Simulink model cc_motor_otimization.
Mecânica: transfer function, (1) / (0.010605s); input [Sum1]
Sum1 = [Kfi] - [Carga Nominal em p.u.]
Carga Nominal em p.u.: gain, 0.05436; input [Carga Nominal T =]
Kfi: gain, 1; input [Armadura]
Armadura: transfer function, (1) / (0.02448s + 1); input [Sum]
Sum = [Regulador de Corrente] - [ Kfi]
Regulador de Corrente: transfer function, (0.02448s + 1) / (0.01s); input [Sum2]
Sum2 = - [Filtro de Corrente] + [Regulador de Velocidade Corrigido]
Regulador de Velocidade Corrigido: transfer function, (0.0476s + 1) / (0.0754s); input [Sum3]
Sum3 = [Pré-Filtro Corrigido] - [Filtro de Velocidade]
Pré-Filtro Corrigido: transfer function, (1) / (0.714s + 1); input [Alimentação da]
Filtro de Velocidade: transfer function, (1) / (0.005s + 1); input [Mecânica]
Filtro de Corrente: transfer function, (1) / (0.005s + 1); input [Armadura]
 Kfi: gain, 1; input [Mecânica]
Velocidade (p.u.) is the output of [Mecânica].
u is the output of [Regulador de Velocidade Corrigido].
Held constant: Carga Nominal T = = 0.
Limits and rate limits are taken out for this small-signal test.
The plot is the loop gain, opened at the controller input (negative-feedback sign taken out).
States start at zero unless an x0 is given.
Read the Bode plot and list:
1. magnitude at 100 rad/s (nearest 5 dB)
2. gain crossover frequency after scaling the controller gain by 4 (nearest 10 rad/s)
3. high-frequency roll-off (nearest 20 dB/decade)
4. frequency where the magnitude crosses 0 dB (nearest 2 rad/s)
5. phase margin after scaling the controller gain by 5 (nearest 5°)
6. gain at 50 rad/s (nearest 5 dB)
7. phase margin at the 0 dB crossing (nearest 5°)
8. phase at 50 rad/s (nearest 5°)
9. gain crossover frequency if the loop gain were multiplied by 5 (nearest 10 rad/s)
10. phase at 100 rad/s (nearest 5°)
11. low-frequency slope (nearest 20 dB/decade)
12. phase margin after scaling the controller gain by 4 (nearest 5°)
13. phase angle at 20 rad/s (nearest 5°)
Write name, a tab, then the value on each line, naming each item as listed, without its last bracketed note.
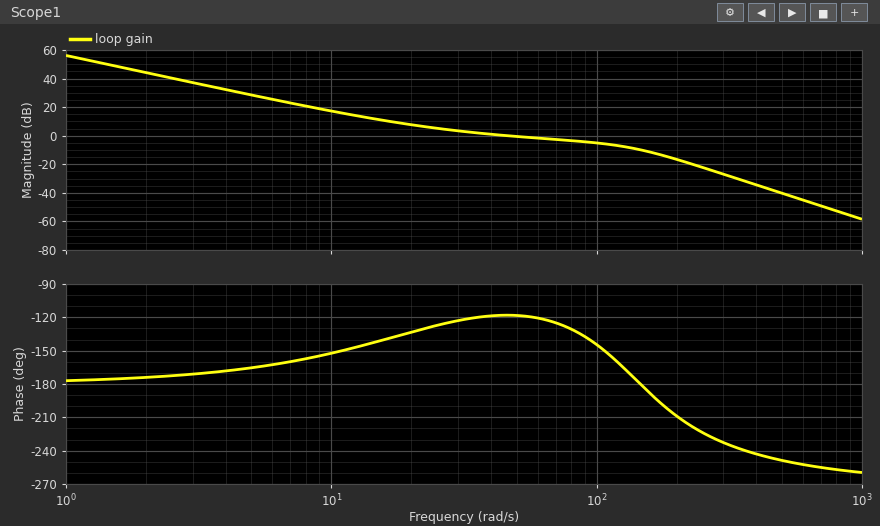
magnitude at 100 rad/s	-5 dB
gain crossover frequency after scaling the controller gain by 4	160 rad/s
high-frequency roll-off	-60 dB/decade
frequency where the magnitude crosses 0 dB	46 rad/s
phase margin after scaling the controller gain by 5	-20°
gain at 50 rad/s	0 dB
phase margin at the 0 dB crossing	60°
phase at 50 rad/s	-120°
gain crossover frequency if the loop gain were multiplied by 5	180 rad/s
phase at 100 rad/s	-145°
low-frequency slope	-40 dB/decade
phase margin after scaling the controller gain by 4	-10°
phase angle at 20 rad/s	-135°
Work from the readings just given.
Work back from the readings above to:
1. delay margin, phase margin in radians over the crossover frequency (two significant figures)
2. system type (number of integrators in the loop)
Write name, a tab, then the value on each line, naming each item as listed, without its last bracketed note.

delay margin, phase margin in radians over the crossover frequency	0.023 s
system type	2
